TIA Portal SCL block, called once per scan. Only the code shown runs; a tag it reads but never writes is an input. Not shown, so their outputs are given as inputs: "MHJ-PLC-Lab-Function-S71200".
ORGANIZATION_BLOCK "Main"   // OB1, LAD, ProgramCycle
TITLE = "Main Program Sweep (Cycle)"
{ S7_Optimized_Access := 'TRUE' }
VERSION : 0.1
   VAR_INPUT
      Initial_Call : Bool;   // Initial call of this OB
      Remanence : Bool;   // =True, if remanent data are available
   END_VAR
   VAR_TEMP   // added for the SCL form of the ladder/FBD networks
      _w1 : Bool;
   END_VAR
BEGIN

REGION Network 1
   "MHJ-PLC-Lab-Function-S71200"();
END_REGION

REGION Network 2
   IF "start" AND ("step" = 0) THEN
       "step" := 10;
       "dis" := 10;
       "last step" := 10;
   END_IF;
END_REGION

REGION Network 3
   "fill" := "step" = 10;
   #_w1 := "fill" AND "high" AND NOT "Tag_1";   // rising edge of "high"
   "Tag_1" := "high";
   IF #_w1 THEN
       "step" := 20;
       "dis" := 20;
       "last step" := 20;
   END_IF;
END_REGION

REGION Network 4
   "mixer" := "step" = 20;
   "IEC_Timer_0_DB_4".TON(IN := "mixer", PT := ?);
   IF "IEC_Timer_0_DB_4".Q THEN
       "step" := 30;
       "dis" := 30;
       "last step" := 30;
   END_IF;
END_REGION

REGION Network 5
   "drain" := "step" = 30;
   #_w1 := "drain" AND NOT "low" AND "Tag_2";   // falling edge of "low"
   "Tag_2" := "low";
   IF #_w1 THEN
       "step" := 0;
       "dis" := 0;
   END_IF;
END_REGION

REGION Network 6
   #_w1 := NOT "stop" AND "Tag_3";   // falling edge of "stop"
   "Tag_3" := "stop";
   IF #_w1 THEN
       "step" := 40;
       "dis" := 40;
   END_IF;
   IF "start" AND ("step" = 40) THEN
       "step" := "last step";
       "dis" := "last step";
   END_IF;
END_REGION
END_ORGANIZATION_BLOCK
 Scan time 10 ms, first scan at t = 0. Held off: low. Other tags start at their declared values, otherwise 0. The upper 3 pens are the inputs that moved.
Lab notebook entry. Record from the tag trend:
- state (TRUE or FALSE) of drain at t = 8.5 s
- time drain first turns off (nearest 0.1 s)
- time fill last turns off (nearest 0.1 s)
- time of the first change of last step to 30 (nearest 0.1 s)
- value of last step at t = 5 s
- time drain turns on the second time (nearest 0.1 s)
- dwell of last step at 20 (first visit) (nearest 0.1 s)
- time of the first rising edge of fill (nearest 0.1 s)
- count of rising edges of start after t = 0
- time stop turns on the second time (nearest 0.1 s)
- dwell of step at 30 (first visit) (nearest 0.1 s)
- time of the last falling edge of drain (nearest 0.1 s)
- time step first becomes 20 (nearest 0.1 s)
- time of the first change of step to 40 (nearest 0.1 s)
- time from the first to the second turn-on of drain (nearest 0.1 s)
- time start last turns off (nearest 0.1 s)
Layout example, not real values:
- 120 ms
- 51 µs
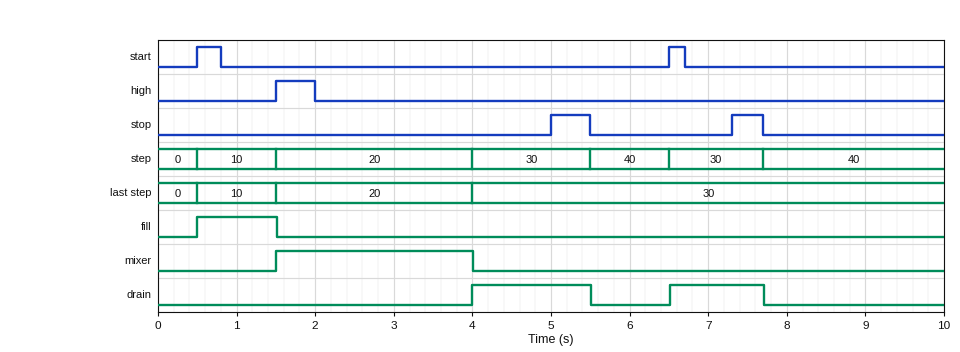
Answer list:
- FALSE
- 5.5 s
- 1.5 s
- 4.0 s
- 30
- 6.5 s
- 2.5 s
- 0.5 s
- 2
- 7.3 s
- 1.5 s
- 7.7 s
- 1.5 s
- 5.5 s
- 2.5 s
- 6.7 s
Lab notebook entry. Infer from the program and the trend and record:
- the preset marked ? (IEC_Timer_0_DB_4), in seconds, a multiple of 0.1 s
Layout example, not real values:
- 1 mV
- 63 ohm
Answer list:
- 2.5 s
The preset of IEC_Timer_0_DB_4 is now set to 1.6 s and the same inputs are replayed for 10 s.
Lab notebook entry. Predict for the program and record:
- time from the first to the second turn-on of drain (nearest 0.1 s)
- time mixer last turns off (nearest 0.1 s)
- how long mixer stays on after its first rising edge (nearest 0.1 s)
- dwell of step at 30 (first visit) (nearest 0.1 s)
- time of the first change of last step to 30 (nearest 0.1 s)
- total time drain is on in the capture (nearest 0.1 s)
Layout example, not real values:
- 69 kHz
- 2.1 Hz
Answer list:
- 3.4 s
- 3.1 s
- 1.6 s
- 2.4 s
- 3.1 s
- 3.6 s
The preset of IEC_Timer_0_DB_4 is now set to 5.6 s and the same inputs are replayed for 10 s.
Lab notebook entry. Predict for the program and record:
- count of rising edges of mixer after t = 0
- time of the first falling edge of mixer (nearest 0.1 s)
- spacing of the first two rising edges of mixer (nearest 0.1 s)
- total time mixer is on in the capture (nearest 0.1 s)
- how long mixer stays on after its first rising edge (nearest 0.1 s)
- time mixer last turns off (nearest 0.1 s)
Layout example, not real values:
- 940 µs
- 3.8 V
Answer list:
- 2
- 5.5 s
- 5.0 s
- 5.2 s
- 4.0 s
- 7.7 s
